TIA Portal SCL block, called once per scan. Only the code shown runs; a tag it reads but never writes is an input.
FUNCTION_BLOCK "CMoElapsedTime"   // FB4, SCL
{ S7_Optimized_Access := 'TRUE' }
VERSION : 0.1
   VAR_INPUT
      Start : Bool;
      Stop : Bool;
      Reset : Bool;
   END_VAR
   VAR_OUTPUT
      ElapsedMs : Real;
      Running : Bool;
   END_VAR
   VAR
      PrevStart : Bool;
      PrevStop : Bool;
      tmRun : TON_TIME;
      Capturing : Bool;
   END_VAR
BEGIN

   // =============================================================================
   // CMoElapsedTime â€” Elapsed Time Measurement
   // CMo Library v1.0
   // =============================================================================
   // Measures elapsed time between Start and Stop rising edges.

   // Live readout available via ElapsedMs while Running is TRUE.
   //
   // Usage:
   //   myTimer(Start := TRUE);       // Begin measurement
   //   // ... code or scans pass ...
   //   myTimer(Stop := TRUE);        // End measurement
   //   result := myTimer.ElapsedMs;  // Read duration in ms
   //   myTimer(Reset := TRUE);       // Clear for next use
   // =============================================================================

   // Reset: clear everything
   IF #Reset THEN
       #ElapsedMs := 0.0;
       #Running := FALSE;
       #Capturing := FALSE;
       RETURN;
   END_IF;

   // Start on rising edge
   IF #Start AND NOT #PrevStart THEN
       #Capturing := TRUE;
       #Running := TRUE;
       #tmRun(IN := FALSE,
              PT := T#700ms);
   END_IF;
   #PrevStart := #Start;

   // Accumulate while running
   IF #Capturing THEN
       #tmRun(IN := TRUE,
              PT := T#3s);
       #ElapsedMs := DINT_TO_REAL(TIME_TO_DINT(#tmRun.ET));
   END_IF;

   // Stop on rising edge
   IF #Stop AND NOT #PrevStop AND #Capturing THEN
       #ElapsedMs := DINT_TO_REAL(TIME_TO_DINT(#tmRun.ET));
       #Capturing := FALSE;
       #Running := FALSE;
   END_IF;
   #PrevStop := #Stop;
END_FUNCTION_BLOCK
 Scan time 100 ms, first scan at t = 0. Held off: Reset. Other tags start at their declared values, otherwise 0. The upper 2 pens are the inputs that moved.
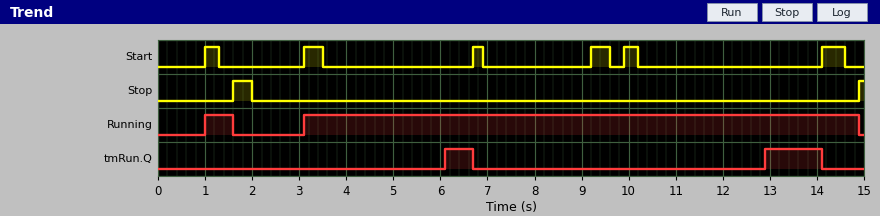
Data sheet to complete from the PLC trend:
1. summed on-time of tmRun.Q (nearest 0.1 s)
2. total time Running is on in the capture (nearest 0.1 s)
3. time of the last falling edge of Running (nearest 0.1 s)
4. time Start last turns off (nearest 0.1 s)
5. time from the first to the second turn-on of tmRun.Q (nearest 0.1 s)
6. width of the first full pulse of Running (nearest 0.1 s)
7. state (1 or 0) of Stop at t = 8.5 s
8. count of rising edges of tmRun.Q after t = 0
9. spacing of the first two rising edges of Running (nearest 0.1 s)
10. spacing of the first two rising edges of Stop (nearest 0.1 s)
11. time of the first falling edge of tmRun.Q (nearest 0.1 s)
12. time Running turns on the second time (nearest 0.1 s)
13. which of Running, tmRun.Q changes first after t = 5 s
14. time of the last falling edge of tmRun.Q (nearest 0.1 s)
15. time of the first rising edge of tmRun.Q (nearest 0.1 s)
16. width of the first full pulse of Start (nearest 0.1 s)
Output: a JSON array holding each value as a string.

["1.8 s", "12.4 s", "14.9 s", "14.6 s", "6.8 s", "0.6 s", "0", "2", "2.1 s", "13.3 s", "6.7 s", "3.1 s", "tmRun.Q", "14.1 s", "6.1 s", "0.3 s"]
